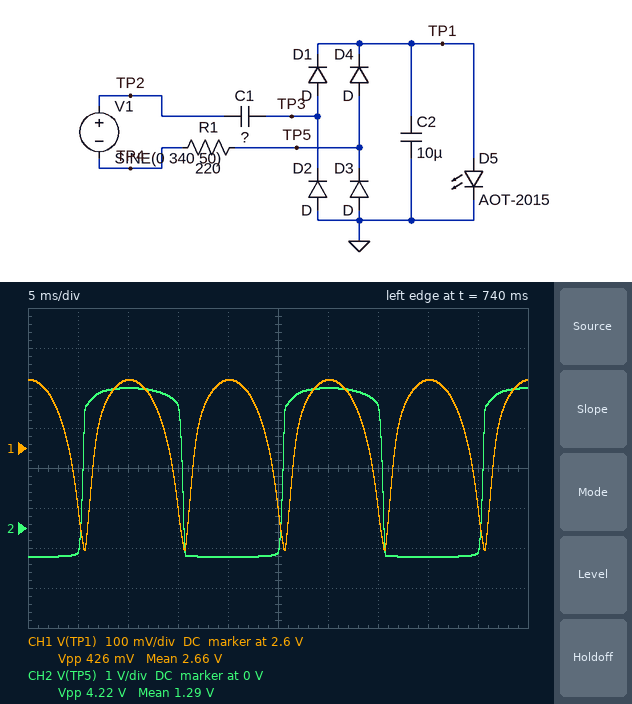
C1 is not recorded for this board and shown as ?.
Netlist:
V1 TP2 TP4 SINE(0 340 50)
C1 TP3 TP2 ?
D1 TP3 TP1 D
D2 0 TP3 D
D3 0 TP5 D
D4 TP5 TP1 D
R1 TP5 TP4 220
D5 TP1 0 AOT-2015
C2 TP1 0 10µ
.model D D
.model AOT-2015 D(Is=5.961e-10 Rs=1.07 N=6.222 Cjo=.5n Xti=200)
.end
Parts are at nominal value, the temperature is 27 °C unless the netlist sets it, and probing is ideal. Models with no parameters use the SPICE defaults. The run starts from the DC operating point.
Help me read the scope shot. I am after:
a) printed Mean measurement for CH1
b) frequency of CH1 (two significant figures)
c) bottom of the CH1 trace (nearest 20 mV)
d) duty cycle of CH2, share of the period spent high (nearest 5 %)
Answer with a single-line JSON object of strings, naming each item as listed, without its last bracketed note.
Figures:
{"printed Mean measurement for CH1": "2.66 V", "frequency of CH1": "100 Hz", "bottom of the CH1 trace": "2.34 V", "duty cycle of CH2, share of the period spent high": "50 %"}
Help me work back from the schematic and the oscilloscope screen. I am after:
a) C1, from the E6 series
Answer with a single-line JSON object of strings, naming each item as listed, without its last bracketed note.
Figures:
{"C1, from the E6 series": "150 nF"}
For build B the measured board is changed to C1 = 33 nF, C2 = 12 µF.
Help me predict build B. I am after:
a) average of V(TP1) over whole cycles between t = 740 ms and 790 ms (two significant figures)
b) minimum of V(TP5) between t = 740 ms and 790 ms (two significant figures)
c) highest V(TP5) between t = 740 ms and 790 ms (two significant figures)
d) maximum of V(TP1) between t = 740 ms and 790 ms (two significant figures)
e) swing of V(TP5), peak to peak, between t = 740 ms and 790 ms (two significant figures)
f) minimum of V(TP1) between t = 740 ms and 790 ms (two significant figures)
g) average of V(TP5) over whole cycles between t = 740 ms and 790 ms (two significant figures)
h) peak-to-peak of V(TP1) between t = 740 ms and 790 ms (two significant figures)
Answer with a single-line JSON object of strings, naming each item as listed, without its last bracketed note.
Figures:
{"average of V(TP1) over whole cycles between t = 740 ms and 790 ms": "2.4 V", "minimum of V(TP5) between t = 740 ms and 790 ms": "-690 mV", "highest V(TP5) between t = 740 ms and 790 ms": "3.2 V", "maximum of V(TP1) between t = 740 ms and 790 ms": "2.5 V", "swing of V(TP5), peak to peak, between t = 740 ms and 790 ms": "3.9 V", "minimum of V(TP1) between t = 740 ms and 790 ms": "2.3 V", "average of V(TP5) over whole cycles between t = 740 ms and 790 ms": "1.2 V", "peak-to-peak of V(TP1) between t = 740 ms and 790 ms": "230 mV"}
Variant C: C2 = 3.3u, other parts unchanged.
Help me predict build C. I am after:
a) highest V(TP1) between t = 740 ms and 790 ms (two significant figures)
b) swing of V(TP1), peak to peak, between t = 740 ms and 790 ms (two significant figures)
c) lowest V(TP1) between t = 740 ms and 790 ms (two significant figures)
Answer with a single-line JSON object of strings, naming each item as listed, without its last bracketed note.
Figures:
{"highest V(TP1) between t = 740 ms and 790 ms": "2.8 V", "swing of V(TP1), peak to peak, between t = 740 ms and 790 ms": "560 mV", "lowest V(TP1) between t = 740 ms and 790 ms": "2.2 V"}
